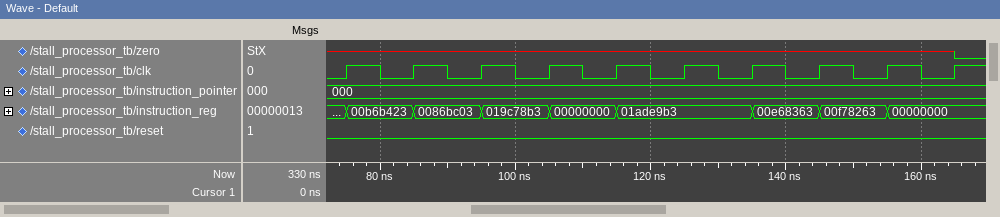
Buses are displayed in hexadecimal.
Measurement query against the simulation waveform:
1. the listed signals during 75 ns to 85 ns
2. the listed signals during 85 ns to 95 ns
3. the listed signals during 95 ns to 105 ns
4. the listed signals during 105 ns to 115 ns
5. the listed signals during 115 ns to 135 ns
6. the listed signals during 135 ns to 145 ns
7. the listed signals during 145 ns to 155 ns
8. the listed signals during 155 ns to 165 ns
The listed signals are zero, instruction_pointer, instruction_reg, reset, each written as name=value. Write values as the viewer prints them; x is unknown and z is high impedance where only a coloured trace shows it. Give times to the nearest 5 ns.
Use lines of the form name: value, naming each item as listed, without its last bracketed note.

the listed signals during 75 ns to 85 ns: zero=x, instruction_pointer=000, instruction_reg=00b6b423, reset=0
the listed signals during 85 ns to 95 ns: zero=x, instruction_pointer=000, instruction_reg=0086bc03, reset=0
the listed signals during 95 ns to 105 ns: zero=x, instruction_pointer=000, instruction_reg=019c78b3, reset=0
the listed signals during 105 ns to 115 ns: zero=x, instruction_pointer=000, instruction_reg=00000000, reset=0
the listed signals during 115 ns to 135 ns: zero=x, instruction_pointer=000, instruction_reg=01ade9b3, reset=0
the listed signals during 135 ns to 145 ns: zero=x, instruction_pointer=000, instruction_reg=00e68363, reset=0
the listed signals during 145 ns to 155 ns: zero=x, instruction_pointer=000, instruction_reg=00f78263, reset=0
the listed signals during 155 ns to 165 ns: zero=x, instruction_pointer=000, instruction_reg=00000000, reset=0
